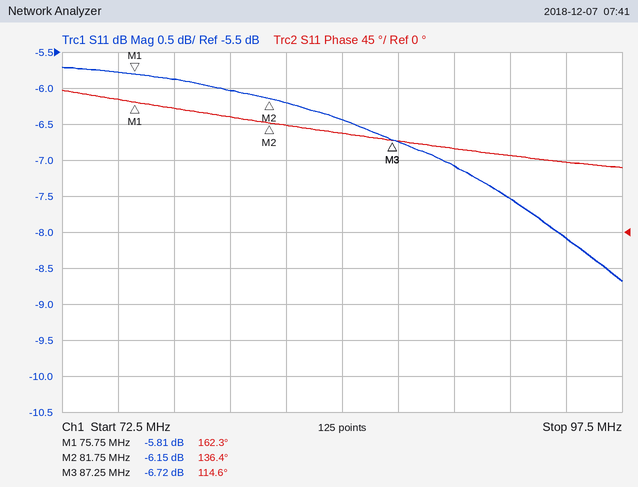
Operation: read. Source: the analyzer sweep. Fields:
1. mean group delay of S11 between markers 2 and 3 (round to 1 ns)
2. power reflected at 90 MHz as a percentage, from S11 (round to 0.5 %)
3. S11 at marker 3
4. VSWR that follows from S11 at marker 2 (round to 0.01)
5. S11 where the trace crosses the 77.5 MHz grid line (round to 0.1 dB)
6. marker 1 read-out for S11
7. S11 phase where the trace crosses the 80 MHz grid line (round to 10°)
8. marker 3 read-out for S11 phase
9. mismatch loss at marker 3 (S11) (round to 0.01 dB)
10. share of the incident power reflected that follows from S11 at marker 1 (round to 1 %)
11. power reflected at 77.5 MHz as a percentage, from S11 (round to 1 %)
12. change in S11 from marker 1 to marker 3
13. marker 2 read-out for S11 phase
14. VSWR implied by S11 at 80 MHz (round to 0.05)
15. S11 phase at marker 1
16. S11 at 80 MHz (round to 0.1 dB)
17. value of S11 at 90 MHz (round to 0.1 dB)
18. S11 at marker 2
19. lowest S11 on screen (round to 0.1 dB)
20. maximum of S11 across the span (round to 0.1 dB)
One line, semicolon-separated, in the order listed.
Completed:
11 ns; 19.5 %; -6.72 dB; 2.94; -5.9 dB; -5.81 dB; 140°; 114.6°; 1.04 dB; 26 %; 26 %; -0.91 dB; 136.4°; 3.00; 162.3°; -6.0 dB; -7.1 dB; -6.15 dB; -8.7 dB; -5.7 dB
